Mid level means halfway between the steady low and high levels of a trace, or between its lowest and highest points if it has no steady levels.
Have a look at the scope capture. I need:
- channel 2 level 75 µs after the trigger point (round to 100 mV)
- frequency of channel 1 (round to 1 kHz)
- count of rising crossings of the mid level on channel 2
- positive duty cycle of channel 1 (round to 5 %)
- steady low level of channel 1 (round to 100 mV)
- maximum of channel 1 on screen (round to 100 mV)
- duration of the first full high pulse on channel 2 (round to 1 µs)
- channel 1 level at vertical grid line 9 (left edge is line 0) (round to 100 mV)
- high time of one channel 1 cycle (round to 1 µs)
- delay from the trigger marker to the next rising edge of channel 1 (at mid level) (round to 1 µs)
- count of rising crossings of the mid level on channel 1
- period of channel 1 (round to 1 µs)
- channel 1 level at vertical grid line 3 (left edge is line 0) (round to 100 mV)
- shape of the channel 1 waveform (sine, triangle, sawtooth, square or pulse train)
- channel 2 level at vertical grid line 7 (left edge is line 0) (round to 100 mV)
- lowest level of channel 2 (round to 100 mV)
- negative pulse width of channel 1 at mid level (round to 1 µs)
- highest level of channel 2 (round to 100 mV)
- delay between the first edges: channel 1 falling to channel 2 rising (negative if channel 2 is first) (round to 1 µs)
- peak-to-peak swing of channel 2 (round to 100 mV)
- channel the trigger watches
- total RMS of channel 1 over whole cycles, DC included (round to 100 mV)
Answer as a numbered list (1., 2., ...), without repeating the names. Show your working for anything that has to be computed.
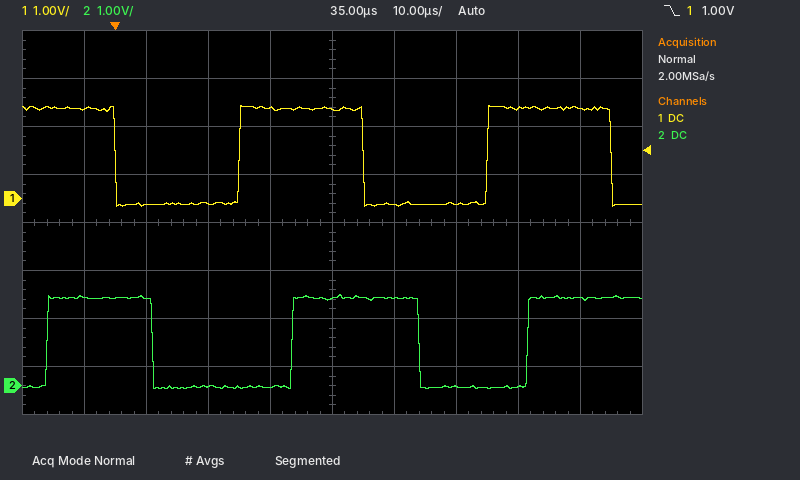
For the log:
1. 1.8 V
2. 1 / 40 µs ≈ 25 kHz
3. 3
4. 20 µs / 40 µs ≈ 50 %
5. -100 mV
6. 1.9 V
7. 17 µs
8. 1.9 V
9. 20 µs
10. 20 µs
11. 2
12. 40 µs
13. -100 mV
14. square
15. 0.0 V
16. -100 mV
17. 20 µs
18. 1.9 V
19. -11 µs
20. 1.9 V − (-100 mV) = 2.0 V
21. channel 1
22. √(0.5 × (1.9 V)² + 0.5 × (-100 mV)²) ≈ 1.3 V
